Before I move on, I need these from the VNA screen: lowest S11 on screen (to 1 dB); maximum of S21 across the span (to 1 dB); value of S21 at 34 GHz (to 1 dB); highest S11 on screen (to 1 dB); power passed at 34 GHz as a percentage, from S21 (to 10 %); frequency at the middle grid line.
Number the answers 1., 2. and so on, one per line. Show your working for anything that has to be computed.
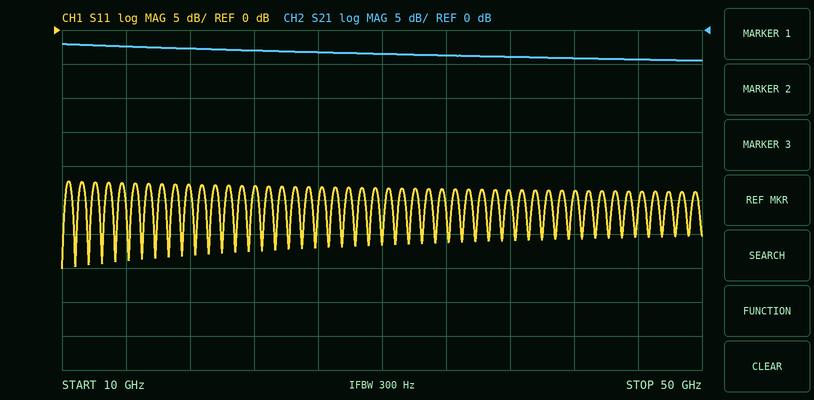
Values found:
1. -35 dB
2. -2 dB
3. -4 dB
4. -22 dB
5. 10^(-4/10) ≈ 40 %
6. 30 GHz
